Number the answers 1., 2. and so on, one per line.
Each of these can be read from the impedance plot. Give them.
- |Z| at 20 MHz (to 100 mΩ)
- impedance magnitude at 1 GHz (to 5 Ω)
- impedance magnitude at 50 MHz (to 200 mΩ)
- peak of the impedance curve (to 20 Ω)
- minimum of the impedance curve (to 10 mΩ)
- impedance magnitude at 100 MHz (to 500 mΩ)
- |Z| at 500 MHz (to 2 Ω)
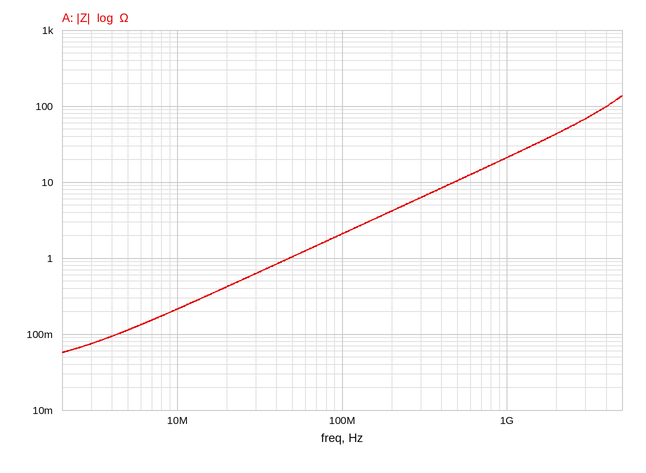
1. 400 mΩ
2. 20 Ω
3. 1.0 Ω
4. 140 Ω
5. 60 mΩ
6. 2.0 Ω
7. 10 Ω
